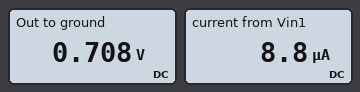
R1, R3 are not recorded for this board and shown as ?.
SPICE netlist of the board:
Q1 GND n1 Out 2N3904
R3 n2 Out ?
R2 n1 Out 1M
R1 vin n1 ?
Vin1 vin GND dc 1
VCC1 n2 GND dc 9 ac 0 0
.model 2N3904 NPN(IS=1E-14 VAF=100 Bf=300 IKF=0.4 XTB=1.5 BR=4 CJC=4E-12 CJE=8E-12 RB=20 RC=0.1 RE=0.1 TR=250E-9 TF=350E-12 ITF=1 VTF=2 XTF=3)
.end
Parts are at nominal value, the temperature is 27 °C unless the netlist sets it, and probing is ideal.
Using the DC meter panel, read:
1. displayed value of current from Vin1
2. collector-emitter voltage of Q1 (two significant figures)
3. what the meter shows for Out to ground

8.8 µA
-710 mV
0.708 V
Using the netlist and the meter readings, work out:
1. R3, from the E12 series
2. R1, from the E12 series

1.8 kΩ
33 kΩ
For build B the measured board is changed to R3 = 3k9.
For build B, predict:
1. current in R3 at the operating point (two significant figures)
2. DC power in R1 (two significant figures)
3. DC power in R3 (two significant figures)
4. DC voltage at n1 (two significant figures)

2.1 mA
3.1 µW
18 mW
680 mV
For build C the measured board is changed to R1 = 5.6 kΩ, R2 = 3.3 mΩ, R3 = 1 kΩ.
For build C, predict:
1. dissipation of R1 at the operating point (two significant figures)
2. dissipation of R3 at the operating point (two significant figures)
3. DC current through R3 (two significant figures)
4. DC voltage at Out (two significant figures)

12 µW
68 mW
8.3 mA
740 mV
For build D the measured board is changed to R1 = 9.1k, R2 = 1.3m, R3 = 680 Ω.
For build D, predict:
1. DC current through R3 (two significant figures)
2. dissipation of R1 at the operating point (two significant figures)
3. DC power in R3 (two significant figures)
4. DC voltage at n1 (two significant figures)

12 mA
6.1 µW
100 mW
760 mV
